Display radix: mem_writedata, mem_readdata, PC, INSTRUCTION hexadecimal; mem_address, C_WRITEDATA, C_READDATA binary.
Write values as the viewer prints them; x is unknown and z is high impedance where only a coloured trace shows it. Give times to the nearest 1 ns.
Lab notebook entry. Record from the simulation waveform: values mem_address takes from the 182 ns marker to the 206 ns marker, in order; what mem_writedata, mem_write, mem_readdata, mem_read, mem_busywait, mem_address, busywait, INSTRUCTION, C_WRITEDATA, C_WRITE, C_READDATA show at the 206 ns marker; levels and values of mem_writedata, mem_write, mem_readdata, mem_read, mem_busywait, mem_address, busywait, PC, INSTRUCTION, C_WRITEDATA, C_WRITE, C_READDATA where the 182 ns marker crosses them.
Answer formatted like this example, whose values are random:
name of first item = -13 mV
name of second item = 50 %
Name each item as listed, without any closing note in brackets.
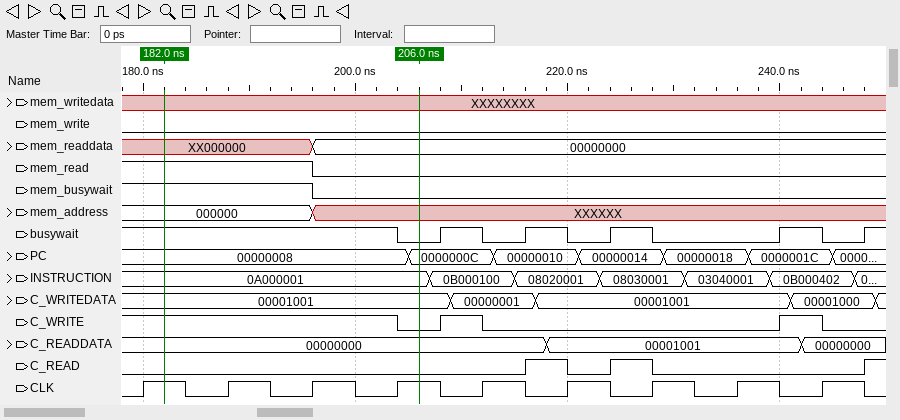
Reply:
values mem_address takes from the 182 ns marker to the 206 ns marker, in order = 000000, XXXXXX
what mem_writedata, mem_write, mem_readdata, mem_read, mem_busywait, mem_address, busywait, INSTRUCTION, C_WRITEDATA, C_WRITE, C_READDATA show at the 206 ns marker = mem_writedata=XXXXXXXX, mem_write=0, mem_readdata=00000000, mem_read=0, mem_busywait=0, mem_address=XXXXXX, busywait=0, INSTRUCTION=0A000001, C_WRITEDATA=00001001, C_WRITE=0, C_READDATA=00000000
levels and values of mem_writedata, mem_write, mem_readdata, mem_read, mem_busywait, mem_address, busywait, PC, INSTRUCTION, C_WRITEDATA, C_WRITE, C_READDATA where the 182 ns marker crosses them = mem_writedata=XXXXXXXX, mem_write=0, mem_readdata=XX000000, mem_read=1, mem_busywait=1, mem_address=000000, busywait=1, PC=00000008, INSTRUCTION=0A000001, C_WRITEDATA=00001001, C_WRITE=1, C_READDATA=00000000
